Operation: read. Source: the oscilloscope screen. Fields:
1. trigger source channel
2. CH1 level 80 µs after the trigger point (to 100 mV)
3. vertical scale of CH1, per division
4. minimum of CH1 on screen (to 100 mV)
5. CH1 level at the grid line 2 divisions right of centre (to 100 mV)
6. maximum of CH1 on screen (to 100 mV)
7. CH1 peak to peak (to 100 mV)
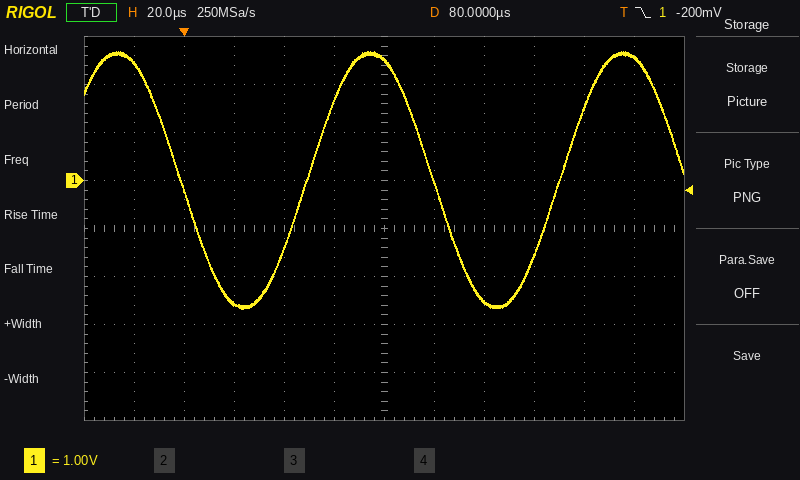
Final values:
CH1
2.5 V
1 V
-2.7 V
-2.5 V
2.7 V
5.4 V
